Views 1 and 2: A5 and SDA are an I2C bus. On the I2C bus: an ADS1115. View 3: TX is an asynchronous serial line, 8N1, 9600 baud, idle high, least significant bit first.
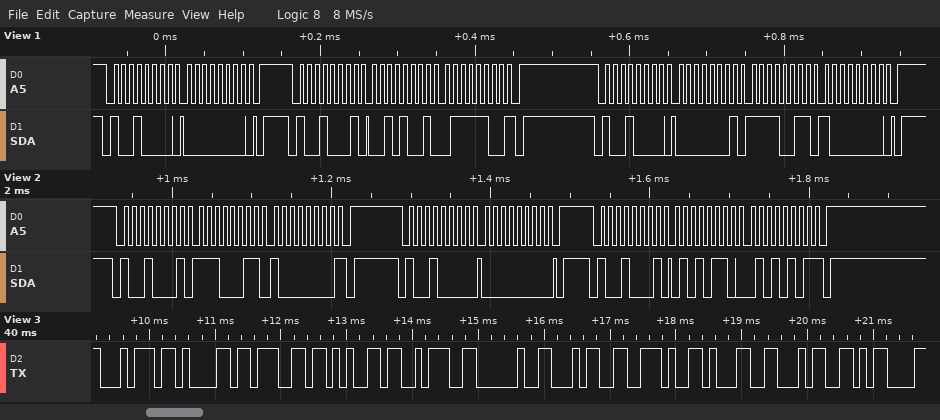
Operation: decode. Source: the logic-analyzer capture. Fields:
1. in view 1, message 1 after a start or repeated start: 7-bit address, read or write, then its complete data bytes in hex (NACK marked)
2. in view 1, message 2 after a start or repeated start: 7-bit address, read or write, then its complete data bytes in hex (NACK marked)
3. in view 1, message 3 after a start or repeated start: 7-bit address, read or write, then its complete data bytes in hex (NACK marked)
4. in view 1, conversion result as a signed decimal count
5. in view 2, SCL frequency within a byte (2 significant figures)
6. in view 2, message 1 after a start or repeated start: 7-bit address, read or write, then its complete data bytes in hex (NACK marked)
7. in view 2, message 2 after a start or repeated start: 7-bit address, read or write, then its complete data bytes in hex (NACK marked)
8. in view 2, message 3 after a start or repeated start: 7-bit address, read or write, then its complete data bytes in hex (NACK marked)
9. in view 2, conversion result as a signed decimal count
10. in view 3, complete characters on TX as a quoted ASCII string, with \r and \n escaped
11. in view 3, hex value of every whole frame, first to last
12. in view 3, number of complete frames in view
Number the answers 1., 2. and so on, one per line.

1. 0x48 write: 00
2. 0x48 read: 29 7C NACK
3. 0x48 write: 01 F3 80
4. 10620
5. 100 kHz
6. 0x48 read: E3 80 NACK
7. 0x48 write: 00
8. 0x48 read: 56 55 NACK
9. 22101
10. "tage: 4.14\r"
11. 74 61 67 65 3A 20 34 2E 31 34 0D
12. 11
